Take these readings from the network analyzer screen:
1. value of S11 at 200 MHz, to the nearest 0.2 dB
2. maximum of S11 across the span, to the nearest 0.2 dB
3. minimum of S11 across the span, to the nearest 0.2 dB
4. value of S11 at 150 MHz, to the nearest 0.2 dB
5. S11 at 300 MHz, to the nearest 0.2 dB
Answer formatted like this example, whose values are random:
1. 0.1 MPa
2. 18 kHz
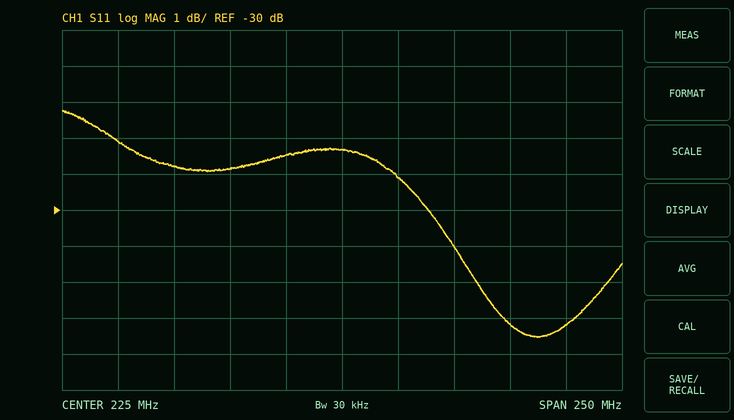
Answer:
1. -28.4 dB
2. -27.2 dB
3. -33.6 dB
4. -28.8 dB
5. -33.2 dB
